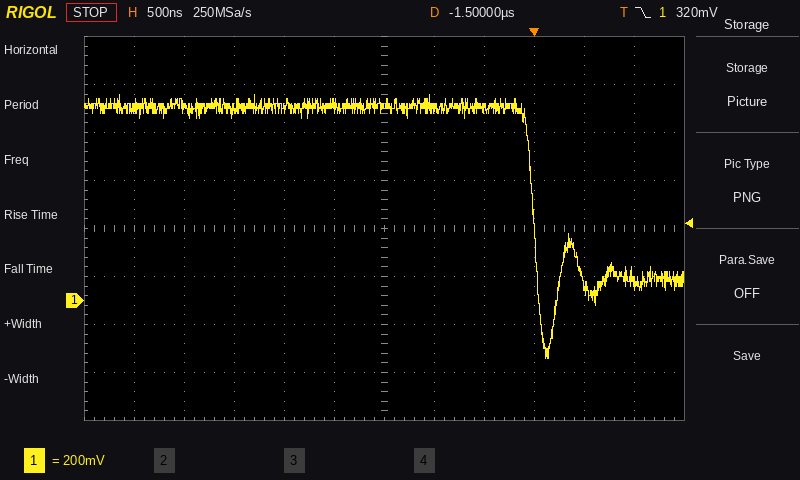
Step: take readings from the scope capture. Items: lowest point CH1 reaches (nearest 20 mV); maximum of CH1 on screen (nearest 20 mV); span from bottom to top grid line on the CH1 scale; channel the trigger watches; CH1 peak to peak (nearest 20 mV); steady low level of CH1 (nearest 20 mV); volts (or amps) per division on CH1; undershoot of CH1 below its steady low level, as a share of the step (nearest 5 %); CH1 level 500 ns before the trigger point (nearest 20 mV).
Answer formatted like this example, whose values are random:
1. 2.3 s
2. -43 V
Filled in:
1. -240 mV
2. 860 mV
3. 1.6 V
4. CH1
5. 1.10 V
6. 100 mV
7. 200 mV
8. 45 %
9. 800 mV
